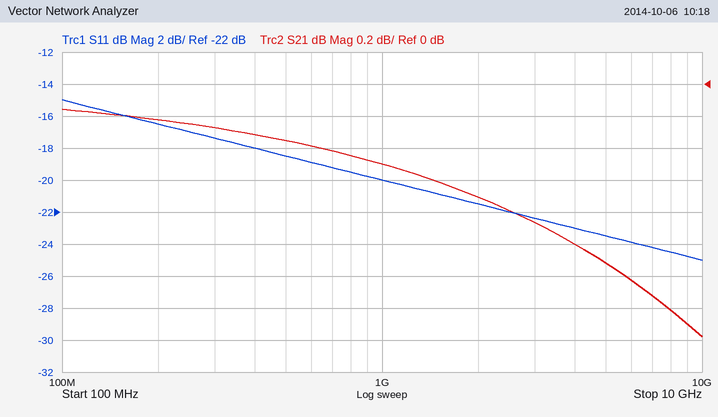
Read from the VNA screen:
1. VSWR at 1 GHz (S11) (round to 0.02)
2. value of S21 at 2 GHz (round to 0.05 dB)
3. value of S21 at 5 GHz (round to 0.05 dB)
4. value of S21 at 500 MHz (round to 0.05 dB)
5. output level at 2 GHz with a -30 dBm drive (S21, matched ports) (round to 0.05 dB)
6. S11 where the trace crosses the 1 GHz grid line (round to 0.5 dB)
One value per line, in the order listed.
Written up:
1.22
-0.70 dB
-1.10 dB
-0.35 dB
-30.70 dBm
-20.0 dB
